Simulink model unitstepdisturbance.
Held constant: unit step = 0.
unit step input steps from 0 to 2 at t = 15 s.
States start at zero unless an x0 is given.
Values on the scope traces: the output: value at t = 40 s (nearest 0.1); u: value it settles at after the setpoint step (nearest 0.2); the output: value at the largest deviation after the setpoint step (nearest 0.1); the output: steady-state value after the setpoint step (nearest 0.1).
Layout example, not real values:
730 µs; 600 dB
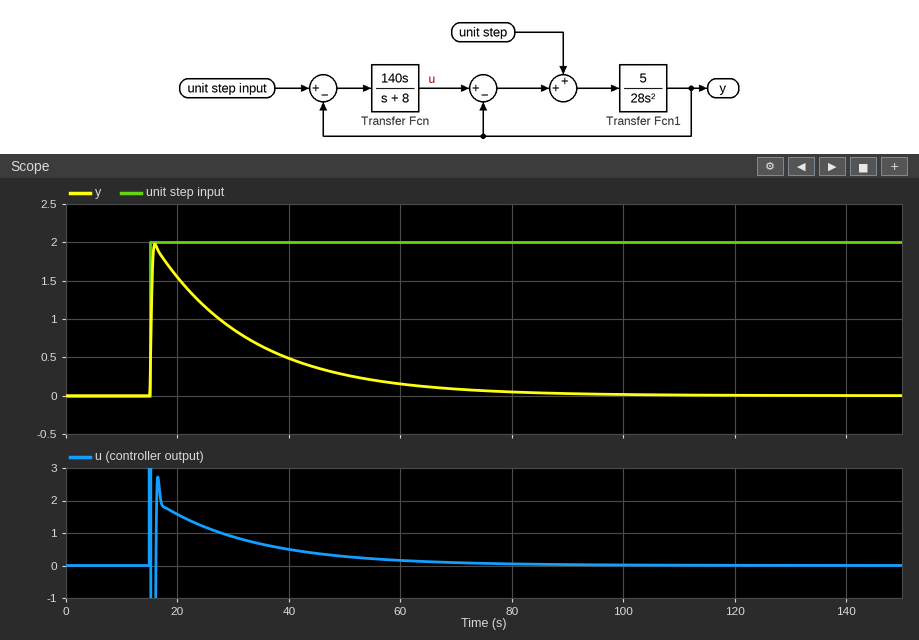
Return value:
0.5; 0.0; 2.0; 0.0
